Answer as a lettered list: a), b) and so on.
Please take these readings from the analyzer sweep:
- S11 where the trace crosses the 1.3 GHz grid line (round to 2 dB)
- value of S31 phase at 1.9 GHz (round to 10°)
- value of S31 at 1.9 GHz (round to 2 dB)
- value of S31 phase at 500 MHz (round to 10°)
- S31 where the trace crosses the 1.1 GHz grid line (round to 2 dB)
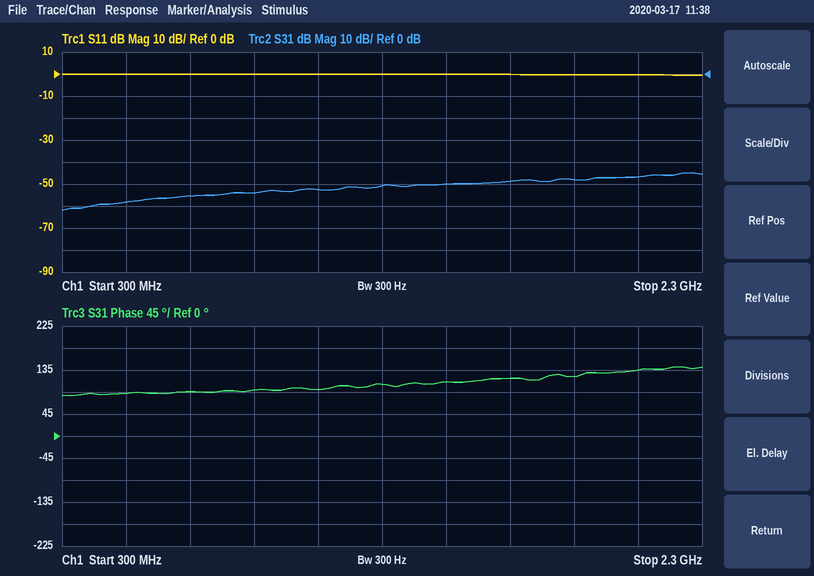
a) 0 dB
b) 120°
c) -48 dB
d) 90°
e) -52 dB
